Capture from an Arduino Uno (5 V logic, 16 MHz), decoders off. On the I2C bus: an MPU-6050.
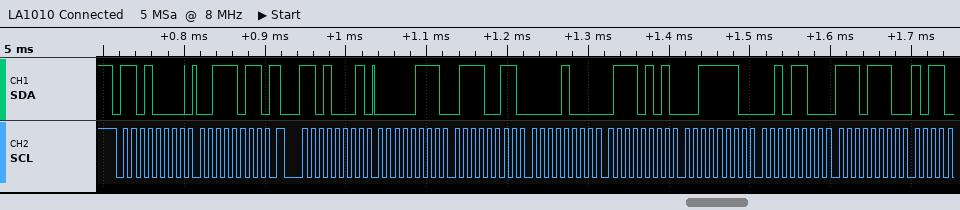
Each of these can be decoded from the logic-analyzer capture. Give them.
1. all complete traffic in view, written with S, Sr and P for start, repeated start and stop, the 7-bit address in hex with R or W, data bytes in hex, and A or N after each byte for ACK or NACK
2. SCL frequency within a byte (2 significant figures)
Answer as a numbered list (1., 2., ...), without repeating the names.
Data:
1. S 68W A 3B A Sr 68R A 07 A 73 A 08 A 75 A 3E A 2C A EE A
2. 100 kHz
